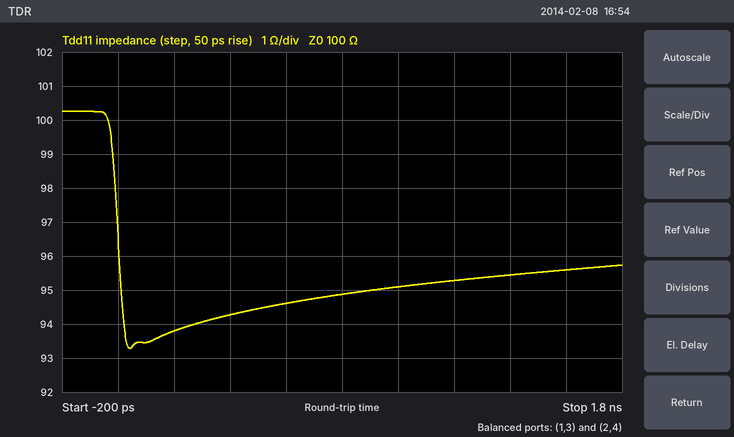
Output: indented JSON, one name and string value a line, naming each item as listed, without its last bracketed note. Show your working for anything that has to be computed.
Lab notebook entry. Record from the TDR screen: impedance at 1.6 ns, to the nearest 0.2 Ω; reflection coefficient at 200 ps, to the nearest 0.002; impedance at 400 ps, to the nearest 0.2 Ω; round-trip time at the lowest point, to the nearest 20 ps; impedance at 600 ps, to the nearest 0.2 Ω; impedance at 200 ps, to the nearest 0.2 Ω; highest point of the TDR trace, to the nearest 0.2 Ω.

{
  "impedance at 1.6 ns, to the nearest 0.2 Ω": "95.6 Ω",
  "reflection coefficient at 200 ps, to the nearest 0.002": "(93.8 − 100)/(93.8 + 100) ≈ -0.032",
  "impedance at 400 ps, to the nearest 0.2 Ω": "94.2 Ω",
  "round-trip time at the lowest point, to the nearest 20 ps": "40 ps",
  "impedance at 600 ps, to the nearest 0.2 Ω": "94.6 Ω",
  "impedance at 200 ps, to the nearest 0.2 Ω": "93.8 Ω",
  "highest point of the TDR trace, to the nearest 0.2 Ω": "100.2 Ω"
}
